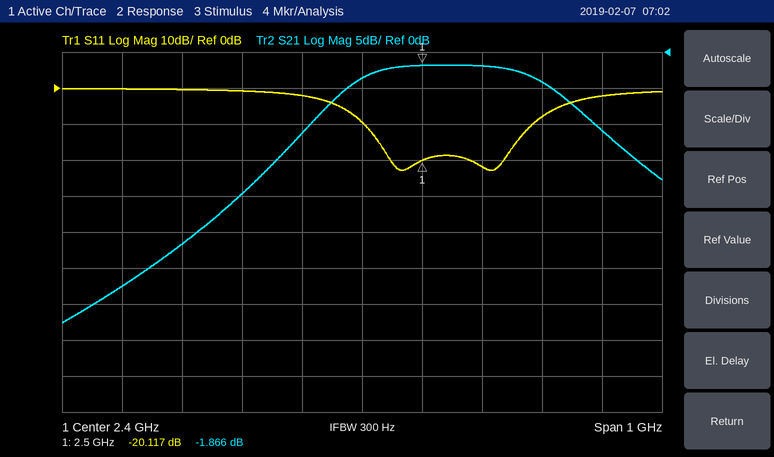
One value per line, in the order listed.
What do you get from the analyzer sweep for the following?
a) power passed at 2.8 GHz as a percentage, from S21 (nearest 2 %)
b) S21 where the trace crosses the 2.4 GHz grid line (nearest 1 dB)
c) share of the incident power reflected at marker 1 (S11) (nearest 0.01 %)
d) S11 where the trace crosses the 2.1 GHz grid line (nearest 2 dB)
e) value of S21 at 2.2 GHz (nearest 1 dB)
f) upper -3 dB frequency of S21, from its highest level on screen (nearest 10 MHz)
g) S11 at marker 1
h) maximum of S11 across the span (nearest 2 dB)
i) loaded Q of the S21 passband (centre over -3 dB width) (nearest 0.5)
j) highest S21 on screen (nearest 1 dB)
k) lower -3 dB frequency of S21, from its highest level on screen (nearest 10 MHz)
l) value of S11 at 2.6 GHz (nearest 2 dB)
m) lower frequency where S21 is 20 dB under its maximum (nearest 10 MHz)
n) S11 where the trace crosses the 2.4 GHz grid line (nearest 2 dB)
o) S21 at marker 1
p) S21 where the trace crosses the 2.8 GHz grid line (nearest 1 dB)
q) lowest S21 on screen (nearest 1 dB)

8 %
-4 dB
0.97 %
0 dB
-20 dB
2.71 GHz
-20.117 dB
0 dB
7.5
-2 dB
2.38 GHz
-22 dB
2.17 GHz
-10 dB
-1.866 dB
-11 dB
-38 dB
